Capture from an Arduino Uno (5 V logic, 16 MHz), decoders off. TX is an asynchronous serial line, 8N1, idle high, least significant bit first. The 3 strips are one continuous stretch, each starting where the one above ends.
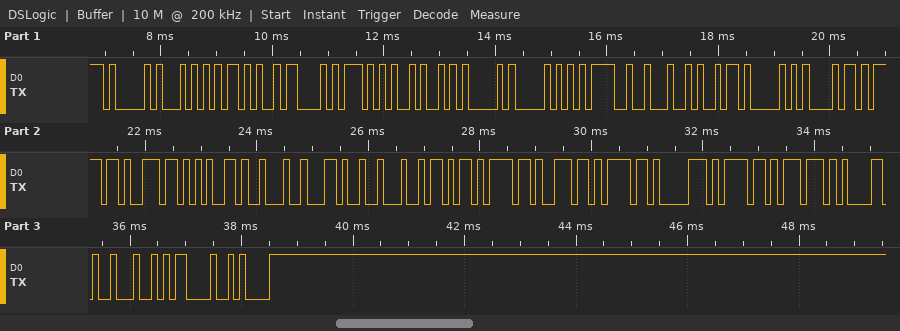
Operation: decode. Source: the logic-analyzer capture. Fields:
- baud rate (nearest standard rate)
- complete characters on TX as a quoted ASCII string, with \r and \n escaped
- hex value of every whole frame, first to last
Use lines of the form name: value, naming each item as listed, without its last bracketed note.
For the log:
baud rate: 9600 baud
complete characters on TX as a quoted ASCII string, with \r and \n escaped: "AT+CWJAP=\"iPhone\",\"konopowa\"\r\n"
hex value of every whole frame, first to last: 41 54 2B 43 57 4A 41 50 3D 22 69 50 68 6F 6E 65 22 2C 22 6B 6F 6E 6F 70 6F 77 61 22 0D 0A
